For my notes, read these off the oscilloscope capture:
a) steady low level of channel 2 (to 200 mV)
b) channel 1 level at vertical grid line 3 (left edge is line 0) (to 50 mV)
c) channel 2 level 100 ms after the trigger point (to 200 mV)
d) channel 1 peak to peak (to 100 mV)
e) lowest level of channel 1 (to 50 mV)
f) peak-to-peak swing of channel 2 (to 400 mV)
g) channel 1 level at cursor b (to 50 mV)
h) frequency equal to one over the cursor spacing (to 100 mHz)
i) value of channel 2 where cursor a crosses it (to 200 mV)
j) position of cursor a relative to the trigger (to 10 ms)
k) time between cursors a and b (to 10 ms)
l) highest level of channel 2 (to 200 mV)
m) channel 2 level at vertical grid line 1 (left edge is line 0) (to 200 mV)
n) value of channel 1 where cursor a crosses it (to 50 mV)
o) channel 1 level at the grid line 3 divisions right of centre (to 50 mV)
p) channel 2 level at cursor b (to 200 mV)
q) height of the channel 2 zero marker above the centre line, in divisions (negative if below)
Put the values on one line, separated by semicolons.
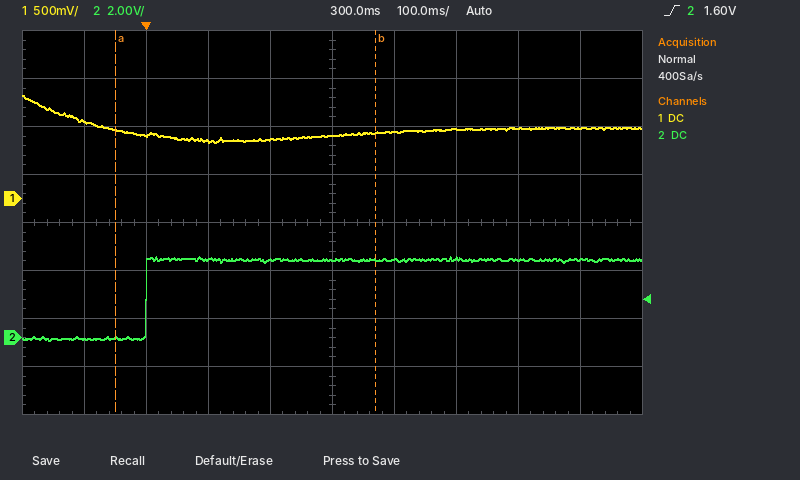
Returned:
0.0 V; 600 mV; 3.2 V; 500 mV; 600 mV; 3.6 V; 700 mV; 2.4 Hz; 0.0 V; -50 ms; 420 ms; 3.4 V; 0.0 V; 700 mV; 750 mV; 3.2 V; -2.4 div
